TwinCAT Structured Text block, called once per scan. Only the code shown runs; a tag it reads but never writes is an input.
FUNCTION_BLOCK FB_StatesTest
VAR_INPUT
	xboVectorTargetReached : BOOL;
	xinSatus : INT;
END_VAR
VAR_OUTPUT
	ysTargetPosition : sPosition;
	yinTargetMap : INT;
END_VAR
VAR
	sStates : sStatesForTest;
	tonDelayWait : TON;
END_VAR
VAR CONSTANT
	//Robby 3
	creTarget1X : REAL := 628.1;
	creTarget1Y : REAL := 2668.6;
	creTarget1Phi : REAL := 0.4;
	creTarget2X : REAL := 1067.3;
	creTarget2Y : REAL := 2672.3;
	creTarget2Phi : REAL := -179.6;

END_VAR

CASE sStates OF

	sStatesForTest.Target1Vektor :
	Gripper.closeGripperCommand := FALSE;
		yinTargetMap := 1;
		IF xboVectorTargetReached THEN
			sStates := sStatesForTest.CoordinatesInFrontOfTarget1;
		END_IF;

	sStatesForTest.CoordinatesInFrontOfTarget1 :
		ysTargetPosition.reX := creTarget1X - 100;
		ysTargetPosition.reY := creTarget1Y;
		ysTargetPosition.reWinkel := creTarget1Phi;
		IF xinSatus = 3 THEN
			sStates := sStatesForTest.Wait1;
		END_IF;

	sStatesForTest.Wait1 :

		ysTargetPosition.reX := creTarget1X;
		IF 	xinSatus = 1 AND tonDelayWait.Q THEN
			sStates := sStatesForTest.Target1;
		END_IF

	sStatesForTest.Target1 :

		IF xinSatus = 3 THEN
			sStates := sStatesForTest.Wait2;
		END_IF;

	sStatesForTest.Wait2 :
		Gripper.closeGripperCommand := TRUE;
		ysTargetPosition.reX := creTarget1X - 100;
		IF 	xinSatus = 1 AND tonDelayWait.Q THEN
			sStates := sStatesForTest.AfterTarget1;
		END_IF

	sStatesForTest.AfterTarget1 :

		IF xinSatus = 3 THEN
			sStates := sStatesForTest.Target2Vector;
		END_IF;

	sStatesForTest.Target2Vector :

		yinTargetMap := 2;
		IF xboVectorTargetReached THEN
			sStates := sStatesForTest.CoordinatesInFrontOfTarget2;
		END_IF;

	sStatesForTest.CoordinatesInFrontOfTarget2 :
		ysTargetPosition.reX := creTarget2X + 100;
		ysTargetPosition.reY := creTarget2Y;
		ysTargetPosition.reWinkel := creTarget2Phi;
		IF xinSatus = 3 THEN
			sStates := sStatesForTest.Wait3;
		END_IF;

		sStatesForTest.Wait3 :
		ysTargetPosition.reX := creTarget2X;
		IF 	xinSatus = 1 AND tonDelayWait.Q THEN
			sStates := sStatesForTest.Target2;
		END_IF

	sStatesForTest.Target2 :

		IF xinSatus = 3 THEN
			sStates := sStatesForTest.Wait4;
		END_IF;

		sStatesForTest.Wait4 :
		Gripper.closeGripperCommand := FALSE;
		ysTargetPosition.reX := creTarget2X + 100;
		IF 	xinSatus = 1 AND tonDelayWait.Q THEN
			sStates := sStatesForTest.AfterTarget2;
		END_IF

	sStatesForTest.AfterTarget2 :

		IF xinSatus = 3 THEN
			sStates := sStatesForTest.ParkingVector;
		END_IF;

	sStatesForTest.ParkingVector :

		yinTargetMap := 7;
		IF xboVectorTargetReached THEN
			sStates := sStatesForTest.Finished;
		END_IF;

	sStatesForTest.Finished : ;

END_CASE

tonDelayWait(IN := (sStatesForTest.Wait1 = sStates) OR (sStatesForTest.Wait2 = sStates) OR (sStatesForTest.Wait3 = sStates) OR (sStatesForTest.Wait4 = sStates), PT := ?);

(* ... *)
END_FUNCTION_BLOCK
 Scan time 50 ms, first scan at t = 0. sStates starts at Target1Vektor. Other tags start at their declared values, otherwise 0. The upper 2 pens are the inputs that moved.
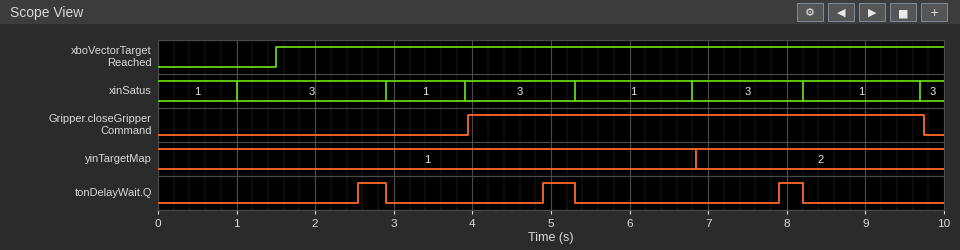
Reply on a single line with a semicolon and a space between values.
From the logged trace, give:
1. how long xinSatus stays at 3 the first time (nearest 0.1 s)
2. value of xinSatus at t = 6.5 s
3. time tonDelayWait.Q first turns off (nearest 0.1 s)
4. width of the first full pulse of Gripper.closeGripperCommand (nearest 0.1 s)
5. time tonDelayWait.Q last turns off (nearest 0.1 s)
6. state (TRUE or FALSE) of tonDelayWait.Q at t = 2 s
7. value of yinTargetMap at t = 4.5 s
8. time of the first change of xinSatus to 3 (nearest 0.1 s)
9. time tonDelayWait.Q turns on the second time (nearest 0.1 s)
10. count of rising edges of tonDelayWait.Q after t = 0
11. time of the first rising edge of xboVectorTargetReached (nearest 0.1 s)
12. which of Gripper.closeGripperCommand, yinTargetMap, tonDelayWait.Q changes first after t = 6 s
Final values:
1.9 s; 1; 2.9 s; 5.8 s; 8.2 s; FALSE; 1; 1.0 s; 4.9 s; 3; 1.5 s; yinTargetMap
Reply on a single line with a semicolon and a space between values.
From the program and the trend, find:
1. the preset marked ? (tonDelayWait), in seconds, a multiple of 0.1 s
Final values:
1.0 s
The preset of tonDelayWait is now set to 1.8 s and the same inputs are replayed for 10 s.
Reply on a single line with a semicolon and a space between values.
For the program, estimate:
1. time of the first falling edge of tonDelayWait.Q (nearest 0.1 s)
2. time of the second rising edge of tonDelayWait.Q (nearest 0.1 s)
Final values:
3.4 s; 5.7 s
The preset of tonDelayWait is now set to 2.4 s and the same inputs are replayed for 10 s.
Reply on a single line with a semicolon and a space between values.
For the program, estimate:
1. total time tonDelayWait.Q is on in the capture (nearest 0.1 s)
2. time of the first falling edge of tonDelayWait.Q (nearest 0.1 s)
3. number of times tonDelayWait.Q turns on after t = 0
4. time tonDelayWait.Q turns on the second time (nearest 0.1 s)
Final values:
1.4 s; 5.3 s; 2; 9.2 s
